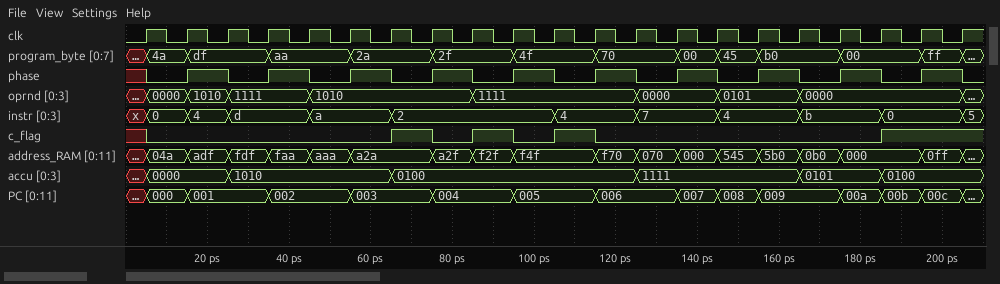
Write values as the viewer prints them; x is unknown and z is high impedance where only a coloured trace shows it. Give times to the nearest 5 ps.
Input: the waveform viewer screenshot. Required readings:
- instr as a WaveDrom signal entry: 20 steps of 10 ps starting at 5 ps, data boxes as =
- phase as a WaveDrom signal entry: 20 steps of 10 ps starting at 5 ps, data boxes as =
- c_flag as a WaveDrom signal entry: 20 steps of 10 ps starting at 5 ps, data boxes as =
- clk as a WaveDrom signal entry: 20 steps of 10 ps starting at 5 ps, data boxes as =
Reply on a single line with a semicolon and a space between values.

{name: 'instr', wave: '===.=.=...=.=.=.=.=.', data: '0 4 d a 2 4 7 4 b 0'}; {name: 'phase', wave: '01010101010101010101'}; {name: 'c_flag', wave: '0.....101010......1.'}; {name: 'clk', wave: 'p...................'}
